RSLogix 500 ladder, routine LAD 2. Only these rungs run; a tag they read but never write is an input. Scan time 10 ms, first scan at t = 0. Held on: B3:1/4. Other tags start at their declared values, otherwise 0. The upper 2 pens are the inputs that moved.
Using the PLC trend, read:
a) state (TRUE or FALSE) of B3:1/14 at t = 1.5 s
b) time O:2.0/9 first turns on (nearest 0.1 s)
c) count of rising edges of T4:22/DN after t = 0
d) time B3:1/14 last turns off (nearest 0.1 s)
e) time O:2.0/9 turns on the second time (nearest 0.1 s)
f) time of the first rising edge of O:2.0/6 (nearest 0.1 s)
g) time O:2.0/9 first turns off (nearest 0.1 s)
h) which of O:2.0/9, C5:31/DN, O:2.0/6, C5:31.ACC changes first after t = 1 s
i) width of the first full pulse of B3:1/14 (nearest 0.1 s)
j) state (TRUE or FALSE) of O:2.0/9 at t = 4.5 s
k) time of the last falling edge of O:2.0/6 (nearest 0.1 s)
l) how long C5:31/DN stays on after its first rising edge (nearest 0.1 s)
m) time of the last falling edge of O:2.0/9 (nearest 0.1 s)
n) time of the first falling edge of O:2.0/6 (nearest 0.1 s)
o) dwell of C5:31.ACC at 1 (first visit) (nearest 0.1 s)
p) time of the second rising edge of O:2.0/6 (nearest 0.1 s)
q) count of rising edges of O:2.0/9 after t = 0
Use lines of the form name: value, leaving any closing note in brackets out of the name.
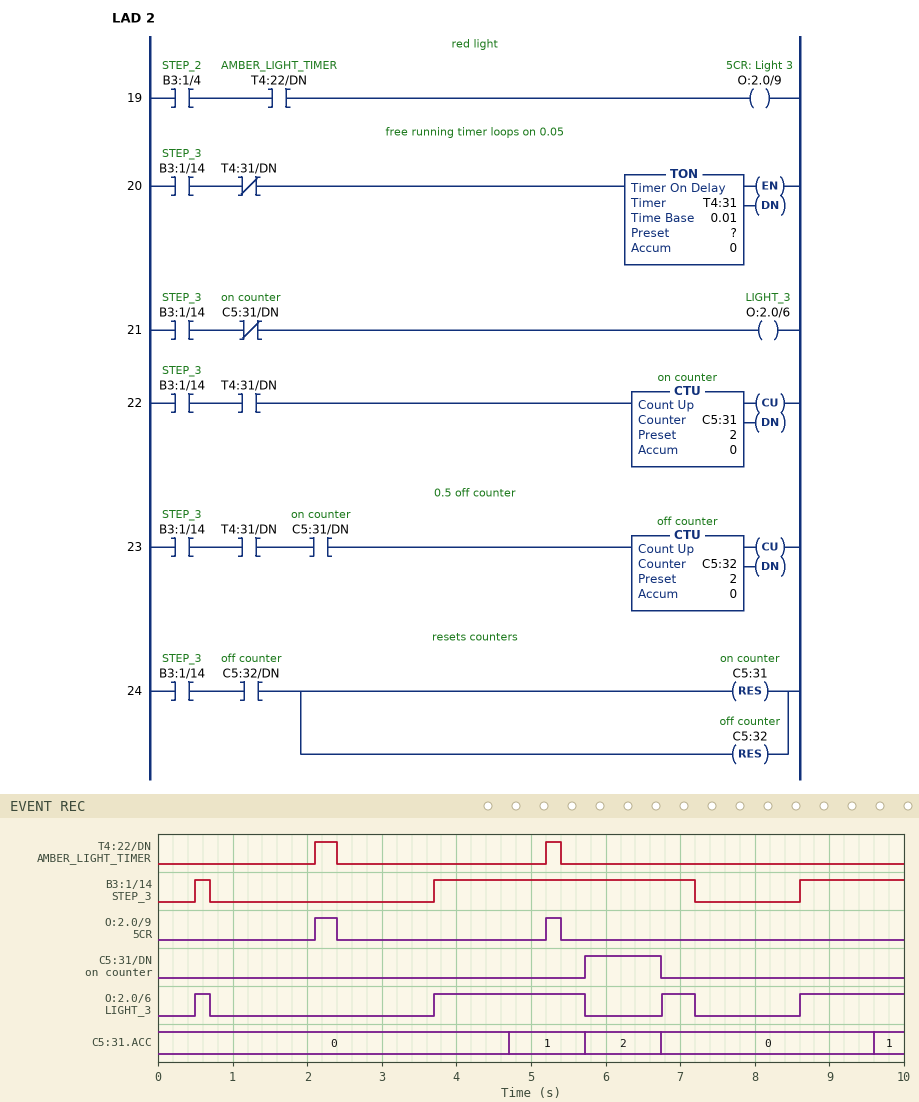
state (TRUE or FALSE) of B3:1/14 at t = 1.5 s: FALSE
time O:2.0/9 first turns on: 2.1 s
count of rising edges of T4:22/DN after t = 0: 2
time B3:1/14 last turns off: 7.2 s
time O:2.0/9 turns on the second time: 5.2 s
time of the first rising edge of O:2.0/6: 0.5 s
time O:2.0/9 first turns off: 2.4 s
which of O:2.0/9, C5:31/DN, O:2.0/6, C5:31.ACC changes first after t = 1 s: O:2.0/9
width of the first full pulse of B3:1/14: 0.2 s
state (TRUE or FALSE) of O:2.0/9 at t = 4.5 s: FALSE
time of the last falling edge of O:2.0/6: 7.2 s
how long C5:31/DN stays on after its first rising edge: 1.0 s
time of the last falling edge of O:2.0/9: 5.4 s
time of the first falling edge of O:2.0/6: 0.7 s
dwell of C5:31.ACC at 1 (first visit): 1.0 s
time of the second rising edge of O:2.0/6: 3.7 s
count of rising edges of O:2.0/9 after t = 0: 2
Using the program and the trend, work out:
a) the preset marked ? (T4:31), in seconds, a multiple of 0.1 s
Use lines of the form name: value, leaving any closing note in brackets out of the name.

the preset marked ? (T4:31), in seconds, a multiple of 0.1 s: 1.0 s
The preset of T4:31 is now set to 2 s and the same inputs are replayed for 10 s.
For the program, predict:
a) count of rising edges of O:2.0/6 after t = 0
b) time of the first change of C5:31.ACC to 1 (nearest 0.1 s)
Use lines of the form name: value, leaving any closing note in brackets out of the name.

count of rising edges of O:2.0/6 after t = 0: 3
time of the first change of C5:31.ACC to 1: 5.7 s
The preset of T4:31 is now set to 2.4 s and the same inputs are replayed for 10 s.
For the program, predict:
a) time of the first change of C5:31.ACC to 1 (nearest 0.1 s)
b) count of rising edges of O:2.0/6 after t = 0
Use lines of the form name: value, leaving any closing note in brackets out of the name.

time of the first change of C5:31.ACC to 1: 6.1 s
count of rising edges of O:2.0/6 after t = 0: 3
